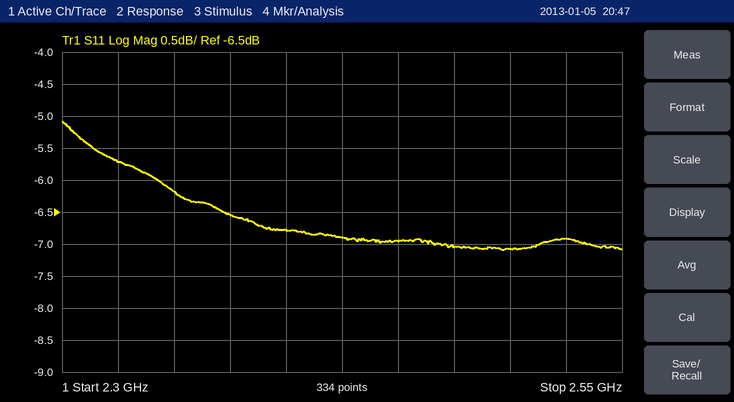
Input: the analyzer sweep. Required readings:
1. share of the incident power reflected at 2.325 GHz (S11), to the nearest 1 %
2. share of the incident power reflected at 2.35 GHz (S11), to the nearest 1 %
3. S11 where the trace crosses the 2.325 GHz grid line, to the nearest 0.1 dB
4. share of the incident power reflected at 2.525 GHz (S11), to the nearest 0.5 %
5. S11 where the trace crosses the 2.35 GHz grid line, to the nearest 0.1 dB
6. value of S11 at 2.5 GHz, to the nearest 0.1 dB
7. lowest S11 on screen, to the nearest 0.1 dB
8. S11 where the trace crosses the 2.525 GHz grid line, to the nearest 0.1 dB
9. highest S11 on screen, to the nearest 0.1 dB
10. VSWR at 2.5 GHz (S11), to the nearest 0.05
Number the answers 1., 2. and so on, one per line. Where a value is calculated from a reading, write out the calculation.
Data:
1. 10^(-5.7/10) ≈ 27 %
2. 10^(-6.2/10) ≈ 24 %
3. -5.7 dB
4. 10^(-6.9/10) ≈ 20.4 %, so 20.5 % to the nearest 0.5 %
5. -6.2 dB
6. -7.1 dB
7. -7.1 dB
8. -6.9 dB
9. -5.1 dB
10. |Γ| = 10^(-7.1/20) = 0.4416; VSWR = (1 + 0.4416)/(1 − 0.4416) ≈ 2.58, so 2.60 to the nearest 0.05
